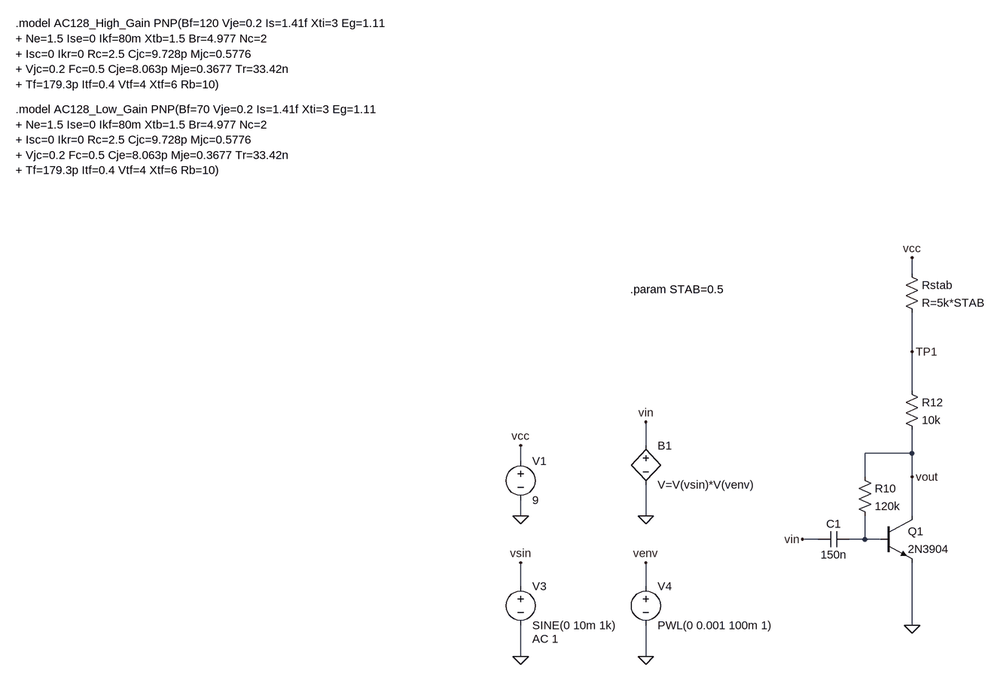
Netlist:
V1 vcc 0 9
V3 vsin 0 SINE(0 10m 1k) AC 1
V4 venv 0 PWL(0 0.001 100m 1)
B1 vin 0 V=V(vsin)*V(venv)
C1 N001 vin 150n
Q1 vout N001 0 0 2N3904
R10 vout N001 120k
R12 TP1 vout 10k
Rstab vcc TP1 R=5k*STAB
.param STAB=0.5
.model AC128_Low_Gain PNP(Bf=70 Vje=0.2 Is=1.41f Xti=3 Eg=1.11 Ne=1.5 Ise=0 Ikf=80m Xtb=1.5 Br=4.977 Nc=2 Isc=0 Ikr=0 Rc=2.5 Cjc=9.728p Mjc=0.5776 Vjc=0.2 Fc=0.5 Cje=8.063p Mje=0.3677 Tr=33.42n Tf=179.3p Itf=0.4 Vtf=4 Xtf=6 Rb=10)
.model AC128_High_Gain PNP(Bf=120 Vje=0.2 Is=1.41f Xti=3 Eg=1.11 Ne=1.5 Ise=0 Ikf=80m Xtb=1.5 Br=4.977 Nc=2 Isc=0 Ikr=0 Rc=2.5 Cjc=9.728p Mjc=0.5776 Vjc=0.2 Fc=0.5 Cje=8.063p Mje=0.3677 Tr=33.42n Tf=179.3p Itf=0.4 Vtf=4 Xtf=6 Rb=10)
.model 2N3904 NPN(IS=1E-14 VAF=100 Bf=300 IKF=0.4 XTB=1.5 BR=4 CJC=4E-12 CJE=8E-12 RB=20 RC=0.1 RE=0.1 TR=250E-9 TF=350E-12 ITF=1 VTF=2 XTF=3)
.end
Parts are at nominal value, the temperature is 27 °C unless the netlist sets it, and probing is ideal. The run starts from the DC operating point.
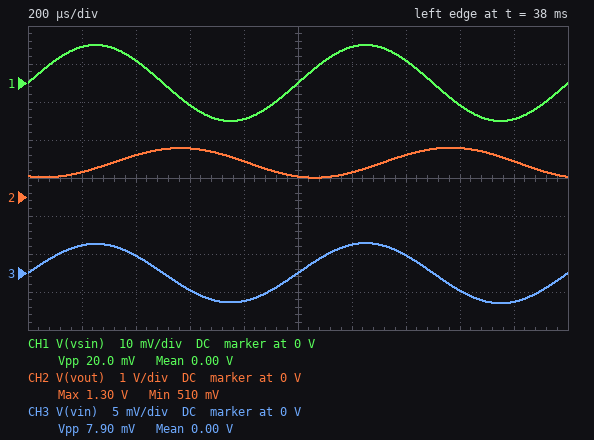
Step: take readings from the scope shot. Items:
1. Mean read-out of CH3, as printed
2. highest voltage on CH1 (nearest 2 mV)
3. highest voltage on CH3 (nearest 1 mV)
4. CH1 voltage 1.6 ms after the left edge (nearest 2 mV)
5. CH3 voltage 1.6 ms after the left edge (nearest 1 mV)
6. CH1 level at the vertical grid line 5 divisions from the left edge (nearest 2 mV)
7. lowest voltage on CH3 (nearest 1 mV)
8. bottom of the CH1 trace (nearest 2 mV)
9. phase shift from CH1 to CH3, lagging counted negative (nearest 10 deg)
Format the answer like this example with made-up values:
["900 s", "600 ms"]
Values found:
["0.00 V", "10 mV", "4 mV", "-6 mV", "-2 mV", "0 V", "-4 mV", "-10 mV", "0 deg"]
